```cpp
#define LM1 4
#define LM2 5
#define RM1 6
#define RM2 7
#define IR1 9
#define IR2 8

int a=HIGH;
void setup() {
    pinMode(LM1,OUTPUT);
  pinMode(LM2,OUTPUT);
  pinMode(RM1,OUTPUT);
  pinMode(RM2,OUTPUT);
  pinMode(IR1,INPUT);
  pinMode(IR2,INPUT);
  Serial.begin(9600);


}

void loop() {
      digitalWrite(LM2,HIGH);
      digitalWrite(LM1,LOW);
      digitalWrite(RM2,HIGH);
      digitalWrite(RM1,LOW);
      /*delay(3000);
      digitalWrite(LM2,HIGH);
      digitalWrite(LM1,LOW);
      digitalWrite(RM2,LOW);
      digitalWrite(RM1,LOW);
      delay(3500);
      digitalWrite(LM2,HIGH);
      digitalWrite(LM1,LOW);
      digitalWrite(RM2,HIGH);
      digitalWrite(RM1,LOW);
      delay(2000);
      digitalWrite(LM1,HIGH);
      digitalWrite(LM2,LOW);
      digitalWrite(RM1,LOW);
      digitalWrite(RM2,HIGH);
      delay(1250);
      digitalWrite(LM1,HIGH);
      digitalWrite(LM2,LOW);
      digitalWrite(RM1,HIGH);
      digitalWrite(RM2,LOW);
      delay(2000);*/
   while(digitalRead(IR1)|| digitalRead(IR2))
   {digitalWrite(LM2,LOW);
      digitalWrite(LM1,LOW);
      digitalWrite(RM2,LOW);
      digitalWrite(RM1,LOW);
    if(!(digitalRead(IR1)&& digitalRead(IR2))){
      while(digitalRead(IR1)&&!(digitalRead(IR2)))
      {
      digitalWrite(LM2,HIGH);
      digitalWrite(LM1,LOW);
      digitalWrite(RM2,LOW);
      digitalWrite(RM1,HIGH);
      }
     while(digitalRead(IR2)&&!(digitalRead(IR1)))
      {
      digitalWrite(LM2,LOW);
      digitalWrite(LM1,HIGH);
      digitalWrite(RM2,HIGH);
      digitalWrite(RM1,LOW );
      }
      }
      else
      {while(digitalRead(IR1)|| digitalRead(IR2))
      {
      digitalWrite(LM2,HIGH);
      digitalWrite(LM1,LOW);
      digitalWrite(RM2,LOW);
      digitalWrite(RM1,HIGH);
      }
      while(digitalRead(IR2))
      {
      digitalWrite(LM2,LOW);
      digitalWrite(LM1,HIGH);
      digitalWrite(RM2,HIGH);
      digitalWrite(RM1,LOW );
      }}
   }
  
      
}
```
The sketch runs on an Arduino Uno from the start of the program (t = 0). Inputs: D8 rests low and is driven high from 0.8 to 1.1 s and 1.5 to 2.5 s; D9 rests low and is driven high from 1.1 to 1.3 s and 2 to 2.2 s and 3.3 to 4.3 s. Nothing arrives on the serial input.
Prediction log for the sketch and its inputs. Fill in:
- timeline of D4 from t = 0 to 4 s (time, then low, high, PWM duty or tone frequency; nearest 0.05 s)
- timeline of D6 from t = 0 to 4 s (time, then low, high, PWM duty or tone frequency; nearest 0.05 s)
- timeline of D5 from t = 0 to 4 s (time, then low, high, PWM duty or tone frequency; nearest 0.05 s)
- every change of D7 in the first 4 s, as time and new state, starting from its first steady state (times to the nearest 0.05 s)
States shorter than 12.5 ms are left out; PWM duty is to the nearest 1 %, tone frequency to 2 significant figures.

0 s low; 0.8 s high; 1.1 s low; 1.5 s high; 2 s low
0 s low; 1.1 s high; 1.3 s low; 2 s high; 2.5 s low; 3.3 s high
0 s high; 0.8 s low; 1.1 s high; 1.5 s low; 2 s high
0 s high; 1.1 s low; 1.3 s high; 2 s low; 2.5 s high; 3.3 s low
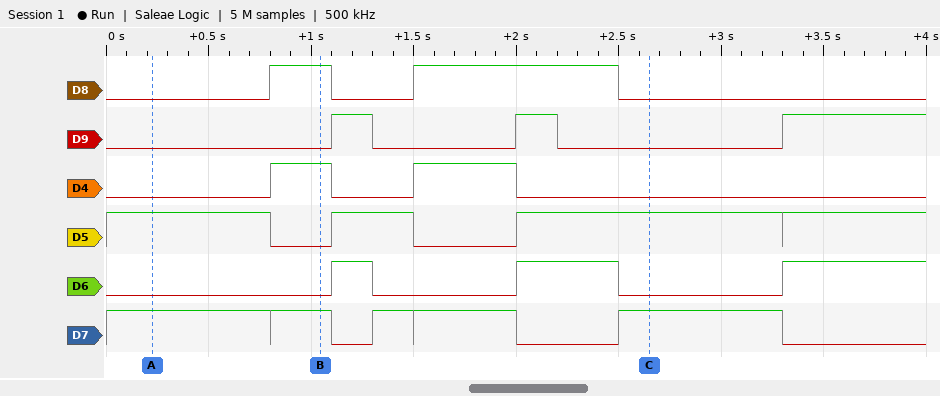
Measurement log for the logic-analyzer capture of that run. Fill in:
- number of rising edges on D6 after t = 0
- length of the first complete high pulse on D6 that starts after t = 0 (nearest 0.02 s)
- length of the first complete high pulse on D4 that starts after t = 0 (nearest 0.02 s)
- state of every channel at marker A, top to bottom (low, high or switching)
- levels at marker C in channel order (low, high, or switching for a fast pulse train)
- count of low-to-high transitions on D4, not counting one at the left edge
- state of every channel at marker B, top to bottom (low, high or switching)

3
0.20 s
0.30 s
D8 low, D9 low, D4 low, D5 high, D6 low, D7 high
D8 low, D9 low, D4 low, D5 high, D6 low, D7 high
2
D8 high, D9 low, D4 high, D5 low, D6 low, D7 high
